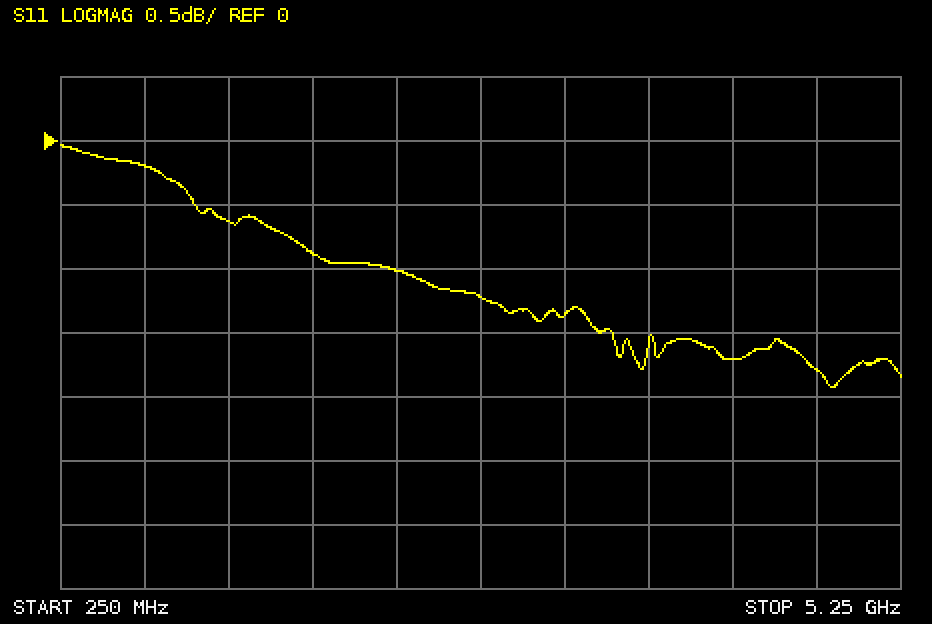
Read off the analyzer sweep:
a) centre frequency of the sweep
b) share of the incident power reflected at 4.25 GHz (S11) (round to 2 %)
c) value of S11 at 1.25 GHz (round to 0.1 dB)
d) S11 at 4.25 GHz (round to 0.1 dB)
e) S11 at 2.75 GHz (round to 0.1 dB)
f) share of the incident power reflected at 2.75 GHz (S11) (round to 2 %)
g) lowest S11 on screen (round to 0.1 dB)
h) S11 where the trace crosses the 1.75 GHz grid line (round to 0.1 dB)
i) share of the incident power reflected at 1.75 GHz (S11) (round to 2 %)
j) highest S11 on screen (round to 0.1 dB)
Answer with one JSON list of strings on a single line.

["2.75 GHz", "68 %", "-0.6 dB", "-1.7 dB", "-1.2 dB", "76 %", "-1.9 dB", "-0.9 dB", "82 %", "0.0 dB"]
